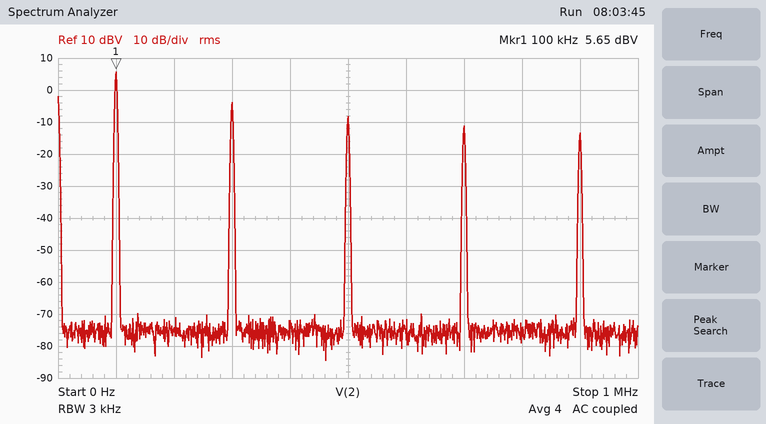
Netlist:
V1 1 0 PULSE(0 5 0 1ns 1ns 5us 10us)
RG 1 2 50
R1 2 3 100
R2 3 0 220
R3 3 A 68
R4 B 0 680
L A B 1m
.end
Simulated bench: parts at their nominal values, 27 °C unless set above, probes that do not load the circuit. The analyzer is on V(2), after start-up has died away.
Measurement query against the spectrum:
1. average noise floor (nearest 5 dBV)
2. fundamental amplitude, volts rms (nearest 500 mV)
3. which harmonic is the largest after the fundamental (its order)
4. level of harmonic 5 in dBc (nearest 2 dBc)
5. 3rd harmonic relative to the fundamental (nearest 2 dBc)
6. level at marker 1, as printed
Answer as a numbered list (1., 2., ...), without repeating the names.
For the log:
1. -75 dBV
2. 2.0 V
3. 3
4. -14 dBc
5. -10 dBc
6. 5.65 dBV
